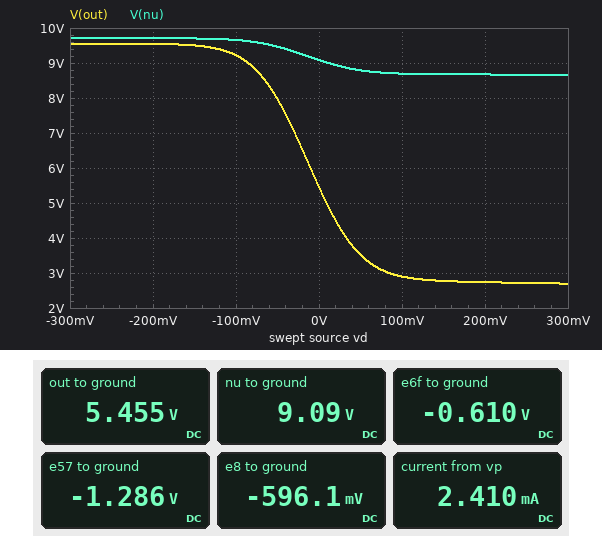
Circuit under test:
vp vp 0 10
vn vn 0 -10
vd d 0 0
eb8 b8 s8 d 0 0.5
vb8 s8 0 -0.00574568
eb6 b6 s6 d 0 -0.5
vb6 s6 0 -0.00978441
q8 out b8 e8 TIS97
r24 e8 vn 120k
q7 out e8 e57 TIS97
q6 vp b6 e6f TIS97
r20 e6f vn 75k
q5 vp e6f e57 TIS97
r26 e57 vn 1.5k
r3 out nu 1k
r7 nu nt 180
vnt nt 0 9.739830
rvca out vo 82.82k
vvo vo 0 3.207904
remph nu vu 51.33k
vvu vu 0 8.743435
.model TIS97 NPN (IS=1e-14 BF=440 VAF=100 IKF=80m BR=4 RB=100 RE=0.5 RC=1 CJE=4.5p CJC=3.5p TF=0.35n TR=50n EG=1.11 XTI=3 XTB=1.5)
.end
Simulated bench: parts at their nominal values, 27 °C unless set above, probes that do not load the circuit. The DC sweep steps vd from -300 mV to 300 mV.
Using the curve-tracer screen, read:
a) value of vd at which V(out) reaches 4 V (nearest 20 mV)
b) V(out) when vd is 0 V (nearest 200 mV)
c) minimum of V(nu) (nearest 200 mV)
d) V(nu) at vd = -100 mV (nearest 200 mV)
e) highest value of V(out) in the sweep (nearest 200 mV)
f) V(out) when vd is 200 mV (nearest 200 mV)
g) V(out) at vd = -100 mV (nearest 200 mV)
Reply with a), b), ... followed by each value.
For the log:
a) 40 mV
b) 5.4 V
c) 8.6 V
d) 9.6 V
e) 9.6 V
f) 2.8 V
g) 9.2 V
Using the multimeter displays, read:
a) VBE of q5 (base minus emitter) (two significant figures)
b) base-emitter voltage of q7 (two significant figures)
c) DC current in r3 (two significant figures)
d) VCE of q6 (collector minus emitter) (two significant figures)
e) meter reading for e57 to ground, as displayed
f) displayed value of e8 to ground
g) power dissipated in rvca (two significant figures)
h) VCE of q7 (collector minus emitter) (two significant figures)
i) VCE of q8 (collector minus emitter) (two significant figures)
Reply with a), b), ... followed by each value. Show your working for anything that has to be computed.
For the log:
a) -610 mV - (-1.286 V) = 680 mV
b) -596.1 mV - (-1.286 V) = 690 mV
c) (9.09 V - 5.455 V) / 1 kΩ = 3.6 mA
d) 10 V - (-610 mV) = 11 V
e) -1.286 V
f) -596.1 mV
g) (5.455 V - 3.208 V)^2 / 82.82 kΩ = 61 µW
h) 5.455 V - (-1.286 V) = 6.7 V
i) 5.455 V - (-596.1 mV) = 6.1 V
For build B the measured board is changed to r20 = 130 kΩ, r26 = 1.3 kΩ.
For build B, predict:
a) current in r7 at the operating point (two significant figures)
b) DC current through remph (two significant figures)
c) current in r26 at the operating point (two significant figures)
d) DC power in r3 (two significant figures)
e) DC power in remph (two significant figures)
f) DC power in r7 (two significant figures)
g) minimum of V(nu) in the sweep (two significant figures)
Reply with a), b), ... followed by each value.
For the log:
a) 3.5 mA
b) 7.3 µA
c) 6.7 mA
d) 12 mW
e) 2.7 µW
f) 2.2 mW
g) 8.5 V
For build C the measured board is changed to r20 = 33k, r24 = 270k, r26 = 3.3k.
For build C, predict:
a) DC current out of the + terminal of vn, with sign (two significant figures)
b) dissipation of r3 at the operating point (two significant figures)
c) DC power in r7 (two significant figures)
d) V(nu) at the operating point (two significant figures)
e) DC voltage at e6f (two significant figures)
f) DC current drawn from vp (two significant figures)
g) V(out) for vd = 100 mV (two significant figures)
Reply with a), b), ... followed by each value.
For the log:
a) -3.0 mA
b) 5.8 mW
c) 1.1 mW
d) 9.3 V
e) -630 mV
f) 600 µA
g) 6.5 V
